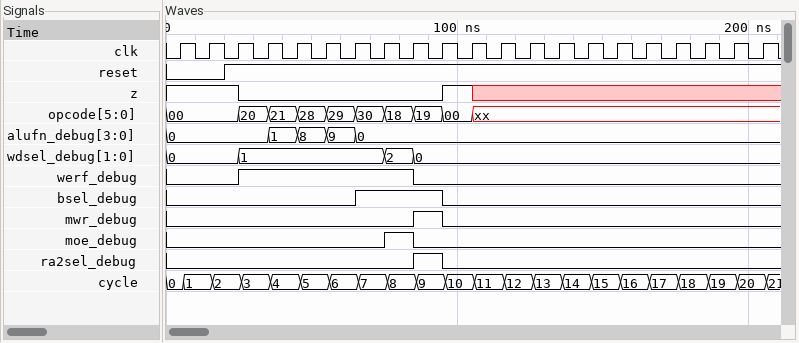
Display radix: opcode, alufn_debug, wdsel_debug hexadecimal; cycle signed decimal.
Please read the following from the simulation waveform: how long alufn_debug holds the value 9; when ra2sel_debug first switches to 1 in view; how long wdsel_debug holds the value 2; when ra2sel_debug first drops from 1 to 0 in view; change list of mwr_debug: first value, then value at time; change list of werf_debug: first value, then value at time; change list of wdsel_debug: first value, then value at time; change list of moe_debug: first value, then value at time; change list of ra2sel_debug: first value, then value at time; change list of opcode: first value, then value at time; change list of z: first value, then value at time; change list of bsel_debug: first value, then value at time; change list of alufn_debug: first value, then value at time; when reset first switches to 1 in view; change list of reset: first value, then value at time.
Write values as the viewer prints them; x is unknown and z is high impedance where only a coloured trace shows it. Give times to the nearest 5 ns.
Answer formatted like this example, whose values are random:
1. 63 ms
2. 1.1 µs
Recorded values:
1. 10 ns
2. 85 ns
3. 10 ns
4. 95 ns
5. 0, 1 at 85 ns, 0 at 95 ns
6. 0, 1 at 25 ns, 0 at 85 ns
7. 0, 1 at 25 ns, 2 at 75 ns, 0 at 85 ns
8. 0, 1 at 75 ns, 0 at 85 ns
9. 0, 1 at 85 ns, 0 at 95 ns
10. 00, 20 at 25 ns, 21 at 35 ns, 28 at 45 ns, 29 at 55 ns, 30 at 65 ns, 18 at 75 ns, 19 at 85 ns, 00 at 95 ns, xx at 105 ns
11. 1, 0 at 25 ns, 1 at 95 ns, x at 105 ns
12. 0, 1 at 65 ns, 0 at 95 ns
13. 0, 1 at 35 ns, 8 at 45 ns, 9 at 55 ns, 0 at 65 ns
14. 20 ns
15. 0, 1 at 20 ns
